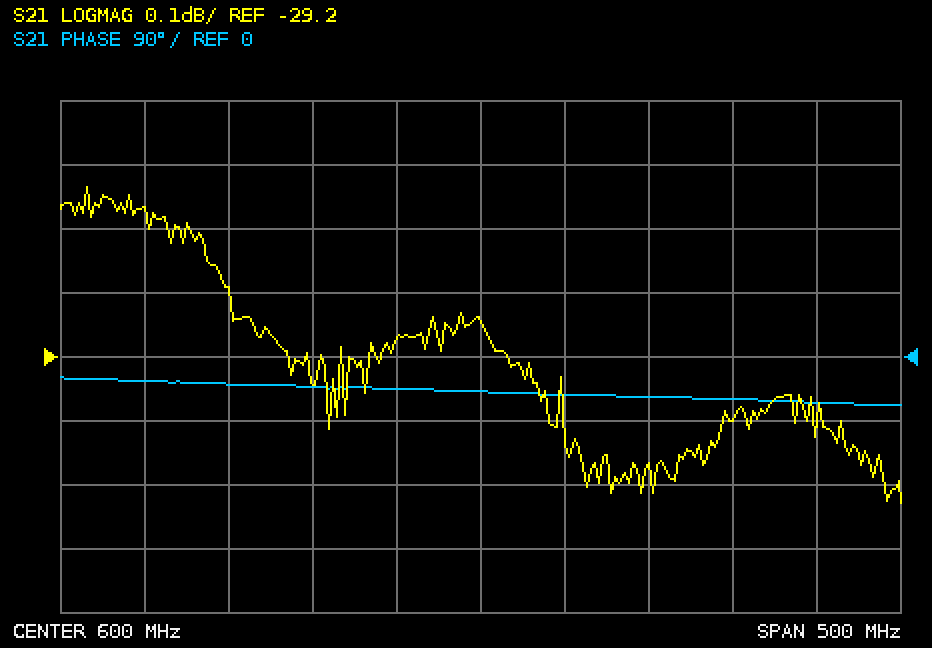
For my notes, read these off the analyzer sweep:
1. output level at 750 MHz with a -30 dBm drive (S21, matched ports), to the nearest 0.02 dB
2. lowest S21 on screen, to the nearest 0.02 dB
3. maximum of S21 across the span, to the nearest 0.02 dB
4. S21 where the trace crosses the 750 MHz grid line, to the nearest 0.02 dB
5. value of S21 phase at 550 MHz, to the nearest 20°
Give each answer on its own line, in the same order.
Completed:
-59.30 dBm
-29.42 dB
-28.94 dB
-29.30 dB
-40°
